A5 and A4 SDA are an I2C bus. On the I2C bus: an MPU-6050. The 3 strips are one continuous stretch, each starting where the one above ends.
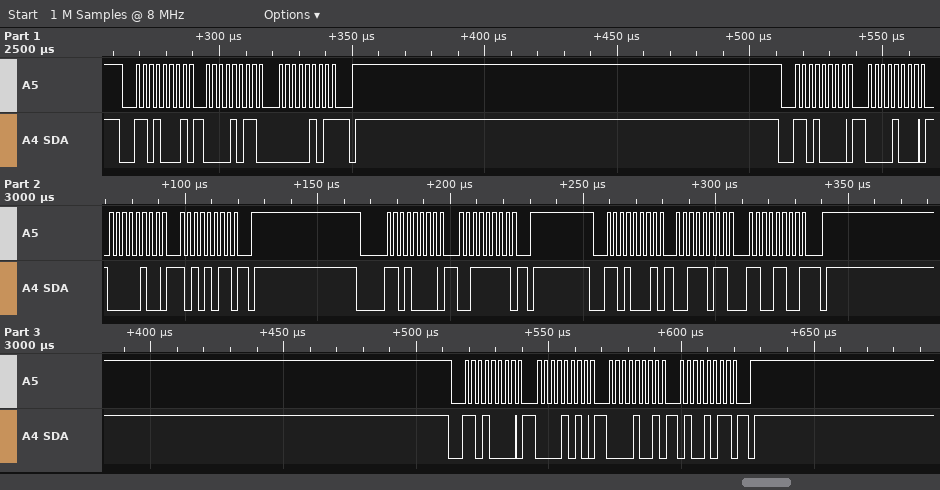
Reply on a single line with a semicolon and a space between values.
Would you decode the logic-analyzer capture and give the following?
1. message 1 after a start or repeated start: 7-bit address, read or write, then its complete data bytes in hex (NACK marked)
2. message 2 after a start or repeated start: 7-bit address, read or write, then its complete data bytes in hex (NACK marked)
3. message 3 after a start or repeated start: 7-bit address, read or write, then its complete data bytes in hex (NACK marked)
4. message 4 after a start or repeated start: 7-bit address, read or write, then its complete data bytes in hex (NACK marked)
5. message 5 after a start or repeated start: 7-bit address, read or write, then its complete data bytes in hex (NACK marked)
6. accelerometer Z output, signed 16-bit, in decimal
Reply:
0x68 read: 0B 05 NACK; 0x68 write: 08 04 AB; 0x68 write: 3F; 0x68 read: 3B CC NACK; 0x68 write: 0A 09 4B; 15308
